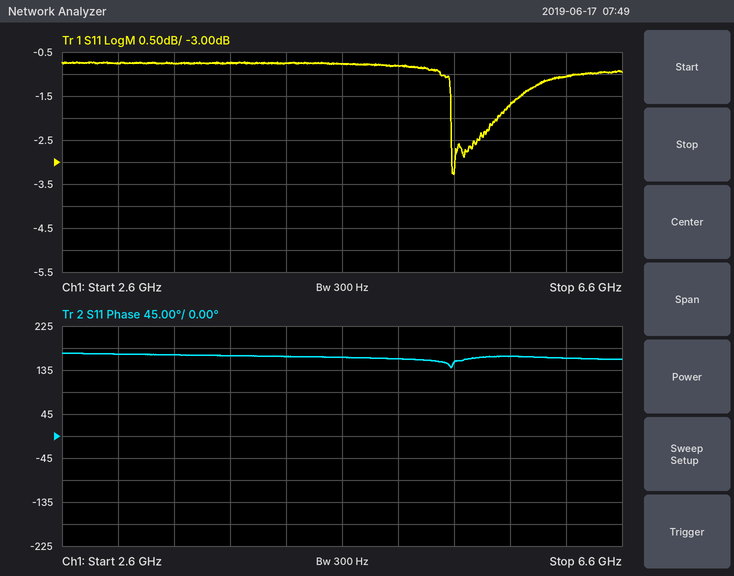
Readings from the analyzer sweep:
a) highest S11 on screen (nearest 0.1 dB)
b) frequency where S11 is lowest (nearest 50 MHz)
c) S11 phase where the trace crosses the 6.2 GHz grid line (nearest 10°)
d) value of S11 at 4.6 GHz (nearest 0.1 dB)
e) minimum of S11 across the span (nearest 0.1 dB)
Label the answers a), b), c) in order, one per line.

a) -0.7 dB
b) 5.40 GHz
c) 160°
d) -0.8 dB
e) -3.3 dB
